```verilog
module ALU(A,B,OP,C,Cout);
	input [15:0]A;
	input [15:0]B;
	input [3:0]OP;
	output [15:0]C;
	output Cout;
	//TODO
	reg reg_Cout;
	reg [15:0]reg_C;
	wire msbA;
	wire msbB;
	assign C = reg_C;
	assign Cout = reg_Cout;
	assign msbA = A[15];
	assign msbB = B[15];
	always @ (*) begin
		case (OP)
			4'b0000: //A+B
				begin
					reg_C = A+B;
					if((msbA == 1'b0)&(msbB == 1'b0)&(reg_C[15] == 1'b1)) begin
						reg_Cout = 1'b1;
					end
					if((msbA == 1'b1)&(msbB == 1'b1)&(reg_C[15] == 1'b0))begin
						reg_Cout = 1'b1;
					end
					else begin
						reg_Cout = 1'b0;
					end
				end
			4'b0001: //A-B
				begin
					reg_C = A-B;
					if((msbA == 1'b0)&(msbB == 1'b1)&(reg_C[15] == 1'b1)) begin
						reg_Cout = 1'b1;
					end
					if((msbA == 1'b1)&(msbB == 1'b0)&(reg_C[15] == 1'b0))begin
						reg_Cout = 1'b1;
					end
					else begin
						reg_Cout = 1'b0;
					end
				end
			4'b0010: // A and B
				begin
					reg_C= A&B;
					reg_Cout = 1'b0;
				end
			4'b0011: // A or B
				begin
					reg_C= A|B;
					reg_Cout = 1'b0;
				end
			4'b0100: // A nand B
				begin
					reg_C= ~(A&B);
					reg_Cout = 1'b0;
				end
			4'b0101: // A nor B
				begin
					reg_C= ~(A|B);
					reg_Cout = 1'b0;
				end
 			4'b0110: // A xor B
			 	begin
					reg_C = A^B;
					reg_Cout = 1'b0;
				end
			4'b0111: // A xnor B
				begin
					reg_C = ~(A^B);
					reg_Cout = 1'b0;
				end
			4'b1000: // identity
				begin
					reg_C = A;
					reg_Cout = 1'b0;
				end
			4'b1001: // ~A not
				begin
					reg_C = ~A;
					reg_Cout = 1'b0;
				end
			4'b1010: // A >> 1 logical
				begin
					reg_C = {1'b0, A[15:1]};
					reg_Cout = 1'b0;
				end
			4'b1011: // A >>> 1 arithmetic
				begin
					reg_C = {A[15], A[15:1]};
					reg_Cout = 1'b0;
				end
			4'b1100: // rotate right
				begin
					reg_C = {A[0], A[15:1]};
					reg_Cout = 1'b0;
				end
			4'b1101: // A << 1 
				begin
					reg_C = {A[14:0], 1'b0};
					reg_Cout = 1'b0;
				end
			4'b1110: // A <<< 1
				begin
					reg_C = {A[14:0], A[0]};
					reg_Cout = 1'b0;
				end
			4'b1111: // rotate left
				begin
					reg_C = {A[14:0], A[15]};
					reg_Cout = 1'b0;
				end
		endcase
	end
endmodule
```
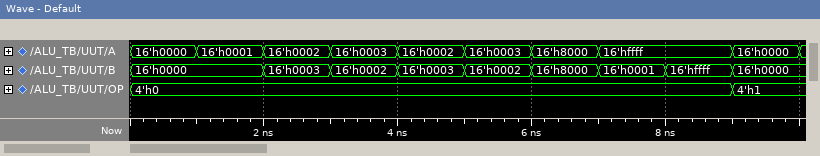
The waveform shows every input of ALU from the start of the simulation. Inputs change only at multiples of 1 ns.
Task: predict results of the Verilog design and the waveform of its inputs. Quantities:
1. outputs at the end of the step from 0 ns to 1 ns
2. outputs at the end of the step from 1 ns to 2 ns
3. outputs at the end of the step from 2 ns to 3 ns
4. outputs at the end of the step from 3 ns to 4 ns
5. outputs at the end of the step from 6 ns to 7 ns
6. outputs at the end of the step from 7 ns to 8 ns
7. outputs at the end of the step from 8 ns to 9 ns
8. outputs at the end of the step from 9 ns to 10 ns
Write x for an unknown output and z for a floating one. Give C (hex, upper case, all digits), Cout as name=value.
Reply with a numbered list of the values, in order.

1. C=0000, Cout=0
2. C=0001, Cout=0
3. C=0005, Cout=0
4. C=0005, Cout=0
5. C=0000, Cout=1
6. C=0000, Cout=0
7. C=FFFE, Cout=0
8. C=0000, Cout=0
